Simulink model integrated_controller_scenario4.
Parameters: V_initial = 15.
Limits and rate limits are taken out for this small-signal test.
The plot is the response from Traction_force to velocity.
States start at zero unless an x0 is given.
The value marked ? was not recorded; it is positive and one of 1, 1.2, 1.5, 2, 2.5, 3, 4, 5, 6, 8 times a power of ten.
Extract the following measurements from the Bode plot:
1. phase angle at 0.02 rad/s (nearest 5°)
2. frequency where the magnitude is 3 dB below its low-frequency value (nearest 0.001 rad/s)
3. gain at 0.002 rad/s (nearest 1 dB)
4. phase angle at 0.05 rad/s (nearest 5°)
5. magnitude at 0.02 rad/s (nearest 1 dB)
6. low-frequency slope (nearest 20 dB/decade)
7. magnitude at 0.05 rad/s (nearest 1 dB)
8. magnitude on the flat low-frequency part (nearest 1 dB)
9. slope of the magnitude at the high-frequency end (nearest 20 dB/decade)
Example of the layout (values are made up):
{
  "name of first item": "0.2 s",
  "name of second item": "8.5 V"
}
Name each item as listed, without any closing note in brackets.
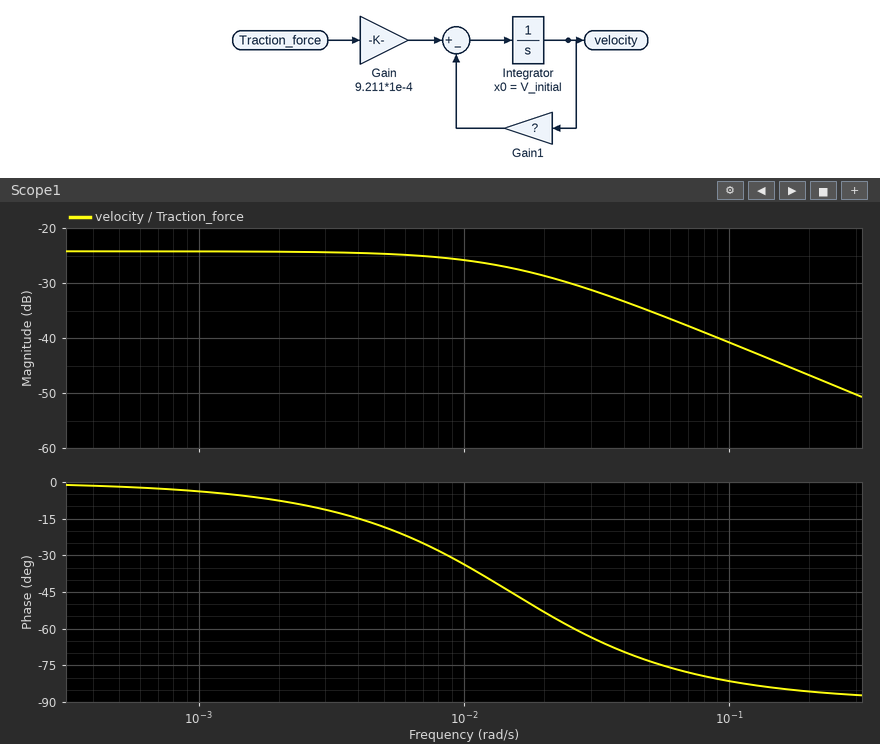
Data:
{
  "phase angle at 0.02 rad/s": "-55°",
  "frequency where the magnitude is 3 dB below its low-frequency value": "0.015 rad/s",
  "gain at 0.002 rad/s": "-24 dB",
  "phase angle at 0.05 rad/s": "-75°",
  "magnitude at 0.02 rad/s": "-29 dB",
  "low-frequency slope": "0 dB/decade",
  "magnitude at 0.05 rad/s": "-35 dB",
  "magnitude on the flat low-frequency part": "-24 dB",
  "slope of the magnitude at the high-frequency end": "-20 dB/decade"
}
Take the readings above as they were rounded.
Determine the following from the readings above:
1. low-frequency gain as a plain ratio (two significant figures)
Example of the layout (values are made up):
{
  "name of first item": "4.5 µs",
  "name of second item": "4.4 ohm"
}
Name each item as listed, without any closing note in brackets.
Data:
{
  "low-frequency gain as a plain ratio": "0.063"
}
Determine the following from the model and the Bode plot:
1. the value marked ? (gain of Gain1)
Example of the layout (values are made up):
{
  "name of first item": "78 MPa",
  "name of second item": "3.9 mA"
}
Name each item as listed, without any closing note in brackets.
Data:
{
  "the value marked ?": "0.015"
}
